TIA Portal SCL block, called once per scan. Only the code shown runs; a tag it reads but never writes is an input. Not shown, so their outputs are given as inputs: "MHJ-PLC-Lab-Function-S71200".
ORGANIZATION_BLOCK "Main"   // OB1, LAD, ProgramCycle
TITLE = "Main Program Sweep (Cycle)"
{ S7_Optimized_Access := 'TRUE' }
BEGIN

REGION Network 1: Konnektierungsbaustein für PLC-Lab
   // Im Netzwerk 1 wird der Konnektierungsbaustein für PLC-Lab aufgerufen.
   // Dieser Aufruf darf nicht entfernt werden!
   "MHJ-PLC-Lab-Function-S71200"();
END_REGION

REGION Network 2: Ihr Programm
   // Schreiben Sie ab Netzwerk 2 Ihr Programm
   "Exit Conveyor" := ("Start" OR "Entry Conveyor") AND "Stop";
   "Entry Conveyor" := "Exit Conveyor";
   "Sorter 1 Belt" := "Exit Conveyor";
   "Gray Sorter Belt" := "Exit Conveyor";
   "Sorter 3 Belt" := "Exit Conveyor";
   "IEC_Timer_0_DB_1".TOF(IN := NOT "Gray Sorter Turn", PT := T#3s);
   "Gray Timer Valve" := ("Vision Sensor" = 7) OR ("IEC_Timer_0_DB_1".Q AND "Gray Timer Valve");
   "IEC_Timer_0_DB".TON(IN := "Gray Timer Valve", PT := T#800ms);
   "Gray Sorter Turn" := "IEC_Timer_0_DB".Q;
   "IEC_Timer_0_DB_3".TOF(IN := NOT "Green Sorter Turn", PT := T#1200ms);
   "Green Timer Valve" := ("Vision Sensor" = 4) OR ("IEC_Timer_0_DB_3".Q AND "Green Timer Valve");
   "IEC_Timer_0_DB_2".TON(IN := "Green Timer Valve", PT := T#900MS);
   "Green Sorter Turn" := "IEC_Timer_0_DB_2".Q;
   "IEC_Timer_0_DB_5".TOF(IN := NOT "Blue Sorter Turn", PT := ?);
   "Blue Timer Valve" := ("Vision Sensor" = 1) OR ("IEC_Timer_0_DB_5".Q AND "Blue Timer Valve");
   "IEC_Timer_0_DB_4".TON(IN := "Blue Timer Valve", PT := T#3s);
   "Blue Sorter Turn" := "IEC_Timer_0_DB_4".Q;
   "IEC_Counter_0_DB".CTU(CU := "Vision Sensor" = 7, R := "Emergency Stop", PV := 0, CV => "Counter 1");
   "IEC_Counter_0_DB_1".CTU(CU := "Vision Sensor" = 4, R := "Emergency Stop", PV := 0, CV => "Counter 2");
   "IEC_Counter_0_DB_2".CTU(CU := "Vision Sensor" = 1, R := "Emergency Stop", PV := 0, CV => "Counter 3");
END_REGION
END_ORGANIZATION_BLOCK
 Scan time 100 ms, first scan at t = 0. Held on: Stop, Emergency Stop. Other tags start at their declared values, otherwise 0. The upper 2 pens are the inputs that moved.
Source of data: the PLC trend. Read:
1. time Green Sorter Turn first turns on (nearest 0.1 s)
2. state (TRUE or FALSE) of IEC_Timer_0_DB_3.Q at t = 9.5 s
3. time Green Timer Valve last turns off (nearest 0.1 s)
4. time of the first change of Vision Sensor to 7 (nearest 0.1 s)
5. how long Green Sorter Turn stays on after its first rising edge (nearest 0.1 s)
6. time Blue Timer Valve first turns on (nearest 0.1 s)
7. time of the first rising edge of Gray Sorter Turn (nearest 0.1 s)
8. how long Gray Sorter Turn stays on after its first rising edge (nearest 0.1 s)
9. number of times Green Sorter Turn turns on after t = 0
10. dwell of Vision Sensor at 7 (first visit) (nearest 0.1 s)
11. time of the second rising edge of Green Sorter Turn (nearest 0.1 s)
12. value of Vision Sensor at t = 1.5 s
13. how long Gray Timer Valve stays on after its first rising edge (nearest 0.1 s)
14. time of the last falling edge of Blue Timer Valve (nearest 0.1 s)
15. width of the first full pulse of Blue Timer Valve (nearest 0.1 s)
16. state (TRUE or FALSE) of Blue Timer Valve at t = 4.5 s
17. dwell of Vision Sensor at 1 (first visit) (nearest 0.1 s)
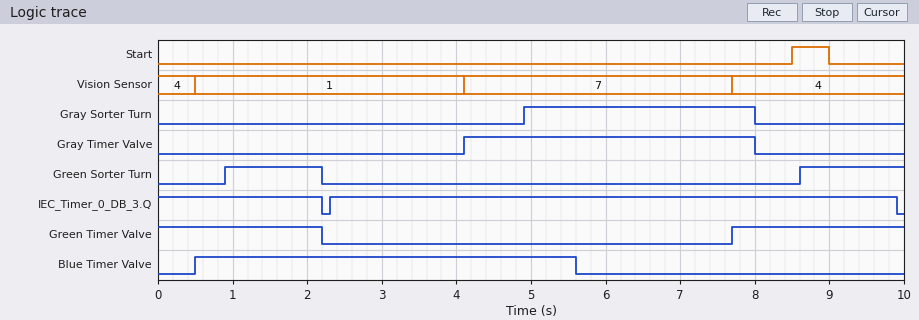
0.9 s
TRUE
2.2 s
4.1 s
1.3 s
0.5 s
4.9 s
3.1 s
2
3.6 s
8.6 s
1
3.9 s
5.6 s
5.1 s
TRUE
3.6 s
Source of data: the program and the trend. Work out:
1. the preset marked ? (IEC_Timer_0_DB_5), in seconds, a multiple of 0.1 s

2.0 s
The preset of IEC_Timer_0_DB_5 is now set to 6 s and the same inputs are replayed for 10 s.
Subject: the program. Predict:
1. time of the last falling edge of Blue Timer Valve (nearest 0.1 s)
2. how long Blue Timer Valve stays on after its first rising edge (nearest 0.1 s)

9.6 s
9.1 s
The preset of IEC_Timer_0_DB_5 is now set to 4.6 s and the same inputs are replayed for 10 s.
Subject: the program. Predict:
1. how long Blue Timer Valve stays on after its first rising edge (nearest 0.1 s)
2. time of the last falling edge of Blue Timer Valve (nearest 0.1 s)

7.7 s
8.2 s
